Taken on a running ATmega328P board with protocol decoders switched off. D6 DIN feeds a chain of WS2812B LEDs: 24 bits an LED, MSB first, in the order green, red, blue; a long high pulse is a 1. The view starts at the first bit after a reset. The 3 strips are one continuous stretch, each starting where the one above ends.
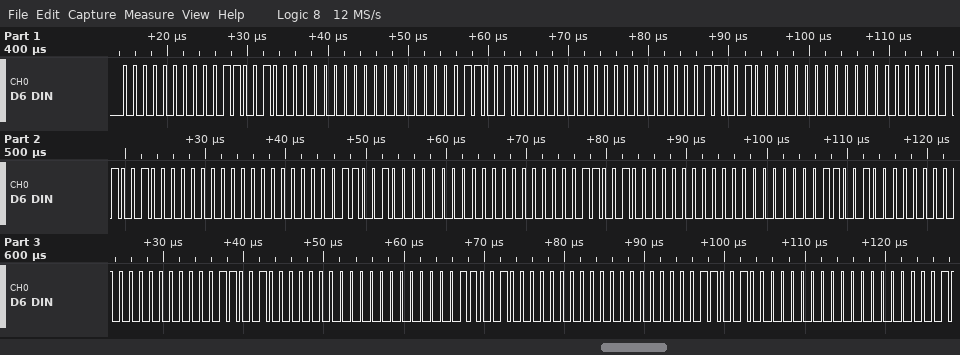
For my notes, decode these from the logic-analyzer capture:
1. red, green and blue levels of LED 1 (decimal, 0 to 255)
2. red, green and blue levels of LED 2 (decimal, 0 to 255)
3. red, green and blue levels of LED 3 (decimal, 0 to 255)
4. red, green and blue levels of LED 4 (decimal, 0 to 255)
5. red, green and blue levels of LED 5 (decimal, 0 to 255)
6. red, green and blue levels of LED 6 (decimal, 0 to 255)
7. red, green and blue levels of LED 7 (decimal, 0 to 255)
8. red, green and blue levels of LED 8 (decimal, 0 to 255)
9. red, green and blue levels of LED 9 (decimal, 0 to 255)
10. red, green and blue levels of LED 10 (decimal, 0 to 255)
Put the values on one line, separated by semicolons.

50, 0, 0; 50, 0, 0; 50, 0, 0; 50, 0, 0; 50, 0, 0; 50, 0, 0; 50, 0, 0; 50, 0, 0; 50, 0, 0; 50, 0, 0
